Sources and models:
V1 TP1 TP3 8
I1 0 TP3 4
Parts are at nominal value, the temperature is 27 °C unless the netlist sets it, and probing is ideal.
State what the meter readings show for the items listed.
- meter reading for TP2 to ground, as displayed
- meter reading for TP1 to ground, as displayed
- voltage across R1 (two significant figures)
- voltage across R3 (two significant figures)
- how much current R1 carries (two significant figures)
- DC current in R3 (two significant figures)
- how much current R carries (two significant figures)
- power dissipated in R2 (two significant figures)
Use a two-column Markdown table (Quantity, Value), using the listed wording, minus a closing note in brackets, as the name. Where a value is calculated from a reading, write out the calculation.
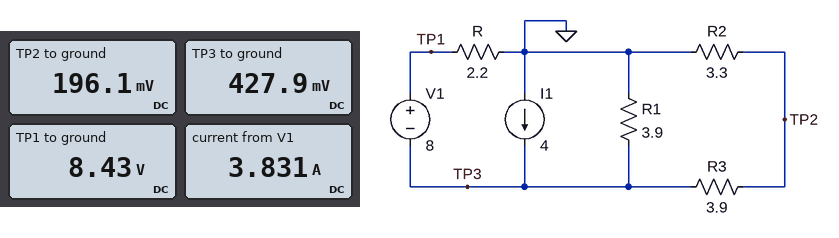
| Quantity | Value |
|---|---|
| meter reading for TP2 to ground, as displayed | 196.1 mV |
| meter reading for TP1 to ground, as displayed | 8.43 V |
| voltage across R1 | 427.9 mV = 430 mV |
| voltage across R3 | 427.9 mV - 196.1 mV = 230 mV |
| how much current R1 carries | (427.9 mV) / 3.9 Ω = 110 mA |
| DC current in R3 | (427.9 mV - 196.1 mV) / 3.9 Ω = 59 mA |
| how much current R carries | (8.43 V) / 2.2 Ω = 3.8 A |
| power dissipated in R2 | (196.1 mV)^2 / 3.3 Ω = 12 mW |
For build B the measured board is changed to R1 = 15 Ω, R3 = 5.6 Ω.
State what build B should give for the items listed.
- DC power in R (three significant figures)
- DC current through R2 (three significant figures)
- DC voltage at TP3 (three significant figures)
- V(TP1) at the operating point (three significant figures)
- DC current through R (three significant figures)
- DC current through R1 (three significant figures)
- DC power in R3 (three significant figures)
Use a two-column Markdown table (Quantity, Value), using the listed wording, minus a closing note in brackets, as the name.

| Quantity | Value |
|---|---|
| DC power in R | 33.4 W |
| DC current through R2 | 64.5 mA |
| DC voltage at TP3 | 574 mV |
| V(TP1) at the operating point | 8.57 V |
| DC current through R | 3.90 A |
| DC current through R1 | 38.3 mA |
| DC power in R3 | 23.3 mW |
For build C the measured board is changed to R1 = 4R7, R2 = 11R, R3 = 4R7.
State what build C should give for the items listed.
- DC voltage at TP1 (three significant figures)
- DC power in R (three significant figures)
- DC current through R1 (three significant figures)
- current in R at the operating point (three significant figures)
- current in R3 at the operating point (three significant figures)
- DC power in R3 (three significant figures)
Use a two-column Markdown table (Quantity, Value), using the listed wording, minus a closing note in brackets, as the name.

| Quantity | Value |
|---|---|
| DC voltage at TP1 | 8.50 V |
| DC power in R | 32.8 W |
| DC current through R1 | 106 mA |
| current in R at the operating point | 3.86 A |
| current in R3 at the operating point | 31.7 mA |
| DC power in R3 | 4.72 mW |
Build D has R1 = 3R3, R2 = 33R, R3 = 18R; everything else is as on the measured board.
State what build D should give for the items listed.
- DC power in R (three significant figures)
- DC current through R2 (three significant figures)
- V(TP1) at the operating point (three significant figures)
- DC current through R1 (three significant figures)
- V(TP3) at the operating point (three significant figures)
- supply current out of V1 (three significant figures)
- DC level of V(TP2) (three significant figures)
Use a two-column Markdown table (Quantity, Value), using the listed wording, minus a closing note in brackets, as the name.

| Quantity | Value |
|---|---|
| DC power in R | 32.6 W |
| DC current through R2 | 9.17 mA |
| V(TP1) at the operating point | 8.47 V |
| DC current through R1 | 142 mA |
| V(TP3) at the operating point | 468 mV |
| supply current out of V1 | 3.85 A |
| DC level of V(TP2) | 303 mV |
